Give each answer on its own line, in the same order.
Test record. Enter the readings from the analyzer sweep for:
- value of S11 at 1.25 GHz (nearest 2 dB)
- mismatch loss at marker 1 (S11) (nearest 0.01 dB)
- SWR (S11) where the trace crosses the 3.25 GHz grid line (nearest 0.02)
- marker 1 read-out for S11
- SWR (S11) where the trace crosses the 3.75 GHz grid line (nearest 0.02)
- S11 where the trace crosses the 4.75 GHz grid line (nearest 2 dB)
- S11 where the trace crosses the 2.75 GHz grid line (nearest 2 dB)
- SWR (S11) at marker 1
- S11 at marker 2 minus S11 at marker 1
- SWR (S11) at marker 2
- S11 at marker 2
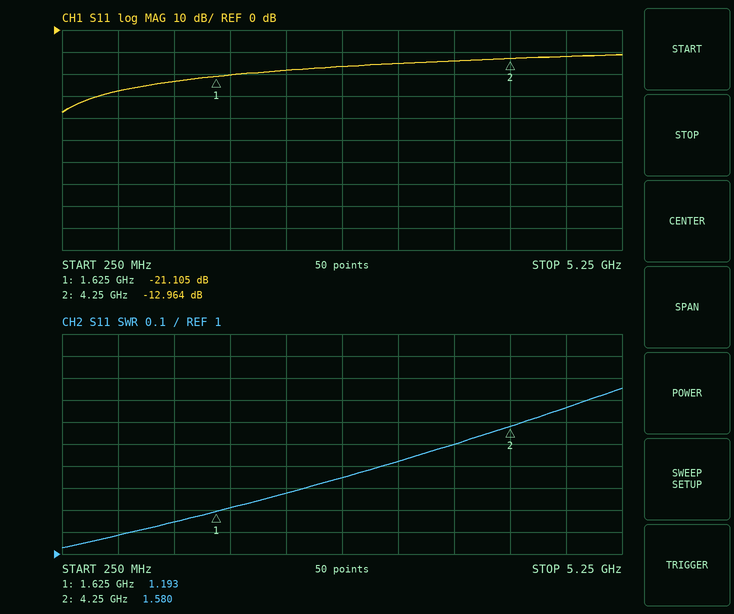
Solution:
-24 dB
0.03 dB
1.42
-21.105 dB
1.50
-12 dB
-16 dB
1.193
8.141 dB
1.580
-12.964 dB
